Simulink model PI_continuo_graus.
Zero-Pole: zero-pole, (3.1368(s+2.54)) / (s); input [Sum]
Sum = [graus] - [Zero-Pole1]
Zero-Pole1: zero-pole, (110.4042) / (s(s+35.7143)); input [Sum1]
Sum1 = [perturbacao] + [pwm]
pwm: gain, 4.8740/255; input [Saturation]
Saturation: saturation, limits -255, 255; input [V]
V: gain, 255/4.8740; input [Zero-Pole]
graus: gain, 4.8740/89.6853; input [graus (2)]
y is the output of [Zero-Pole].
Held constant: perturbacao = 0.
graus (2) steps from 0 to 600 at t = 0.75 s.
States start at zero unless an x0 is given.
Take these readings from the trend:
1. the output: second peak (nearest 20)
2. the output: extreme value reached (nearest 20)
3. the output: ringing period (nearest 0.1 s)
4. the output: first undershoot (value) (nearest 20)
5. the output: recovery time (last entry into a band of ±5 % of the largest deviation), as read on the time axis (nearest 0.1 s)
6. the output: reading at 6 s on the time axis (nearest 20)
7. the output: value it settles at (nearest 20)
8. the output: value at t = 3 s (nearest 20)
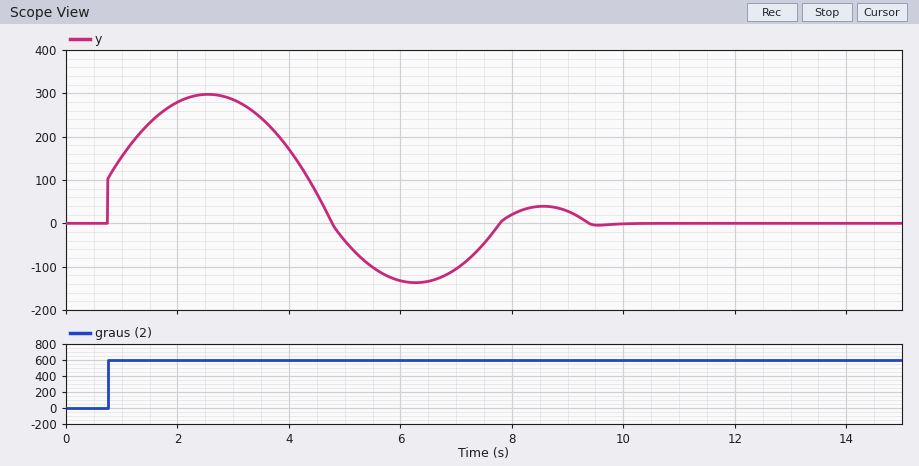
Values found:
40
300
6.0 s
-140
9.2 s
-140
0
280
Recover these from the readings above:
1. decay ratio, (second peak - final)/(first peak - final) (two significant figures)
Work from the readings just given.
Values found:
0.13
